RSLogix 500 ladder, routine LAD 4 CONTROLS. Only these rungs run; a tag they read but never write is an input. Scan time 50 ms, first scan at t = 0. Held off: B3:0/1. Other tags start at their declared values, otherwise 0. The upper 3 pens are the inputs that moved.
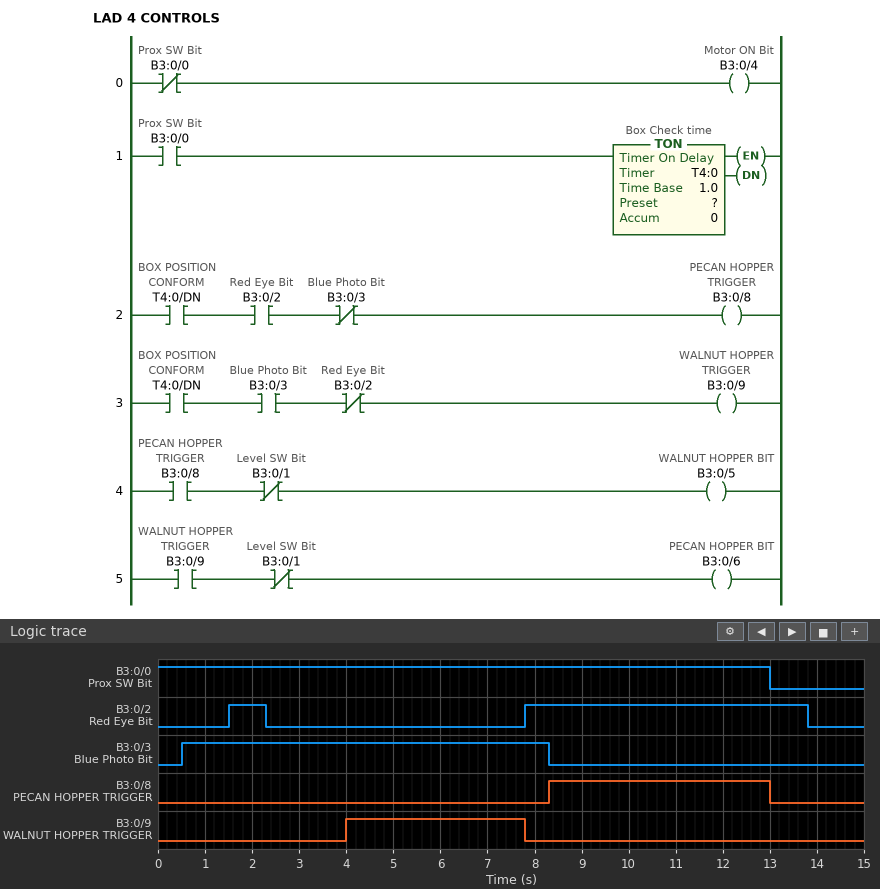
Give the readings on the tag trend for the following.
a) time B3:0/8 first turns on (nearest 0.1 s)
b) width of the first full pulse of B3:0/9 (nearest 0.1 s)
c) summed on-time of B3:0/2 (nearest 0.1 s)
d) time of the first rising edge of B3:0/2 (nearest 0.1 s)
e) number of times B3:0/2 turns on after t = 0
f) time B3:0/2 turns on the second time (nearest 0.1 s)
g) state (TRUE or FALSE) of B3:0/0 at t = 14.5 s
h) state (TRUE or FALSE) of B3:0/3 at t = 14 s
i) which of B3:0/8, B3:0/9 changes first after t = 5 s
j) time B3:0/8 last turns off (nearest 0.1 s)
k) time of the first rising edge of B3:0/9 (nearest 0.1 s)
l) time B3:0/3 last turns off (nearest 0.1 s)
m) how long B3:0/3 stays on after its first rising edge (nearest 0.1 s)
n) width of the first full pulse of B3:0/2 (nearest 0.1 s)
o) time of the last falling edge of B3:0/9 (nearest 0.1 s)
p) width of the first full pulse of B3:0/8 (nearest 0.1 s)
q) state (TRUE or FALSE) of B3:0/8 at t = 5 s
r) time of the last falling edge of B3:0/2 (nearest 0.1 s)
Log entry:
8.3 s
3.8 s
6.8 s
1.5 s
2
7.8 s
FALSE
FALSE
B3:0/9
13.0 s
4.0 s
8.3 s
7.8 s
0.8 s
7.8 s
4.7 s
FALSE
13.8 s
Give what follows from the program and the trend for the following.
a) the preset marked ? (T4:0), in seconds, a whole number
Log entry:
4 s
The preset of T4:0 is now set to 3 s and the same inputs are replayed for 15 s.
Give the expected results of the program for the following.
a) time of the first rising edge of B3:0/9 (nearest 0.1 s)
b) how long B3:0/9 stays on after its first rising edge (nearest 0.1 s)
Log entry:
3.0 s
4.8 s
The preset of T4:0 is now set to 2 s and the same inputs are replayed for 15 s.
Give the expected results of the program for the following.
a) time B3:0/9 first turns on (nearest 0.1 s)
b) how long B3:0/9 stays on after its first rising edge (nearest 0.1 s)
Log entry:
2.3 s
5.5 s
